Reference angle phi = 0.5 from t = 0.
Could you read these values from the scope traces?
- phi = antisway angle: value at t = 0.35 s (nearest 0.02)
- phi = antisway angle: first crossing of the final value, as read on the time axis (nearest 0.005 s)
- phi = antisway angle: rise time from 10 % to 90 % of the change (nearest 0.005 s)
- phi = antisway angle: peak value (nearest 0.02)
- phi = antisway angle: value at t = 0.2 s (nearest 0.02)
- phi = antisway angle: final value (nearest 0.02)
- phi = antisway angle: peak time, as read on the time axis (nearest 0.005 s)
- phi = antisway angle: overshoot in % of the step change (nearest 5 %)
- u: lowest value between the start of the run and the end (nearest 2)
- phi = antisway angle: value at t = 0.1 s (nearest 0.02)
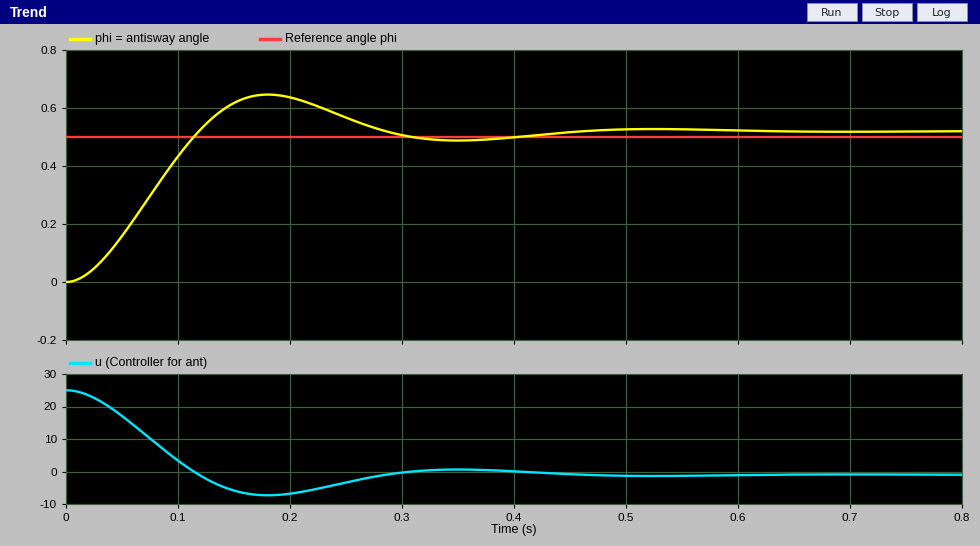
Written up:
0.48
0.120 s
0.080 s
0.64
0.64
0.52
0.180 s
25 %
-8
0.44
